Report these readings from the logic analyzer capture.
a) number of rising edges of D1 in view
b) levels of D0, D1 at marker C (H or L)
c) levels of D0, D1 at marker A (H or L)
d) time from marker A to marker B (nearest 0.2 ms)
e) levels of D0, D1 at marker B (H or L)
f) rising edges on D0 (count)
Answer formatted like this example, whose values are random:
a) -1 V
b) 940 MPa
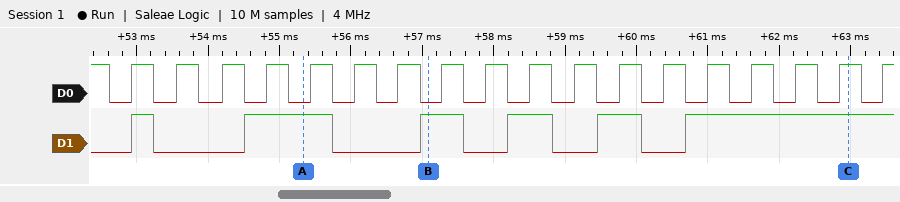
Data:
a) 6
b) D0=H, D1=H
c) D0=L, D1=H
d) 1.8 ms
e) D0=L, D1=H
f) 18
